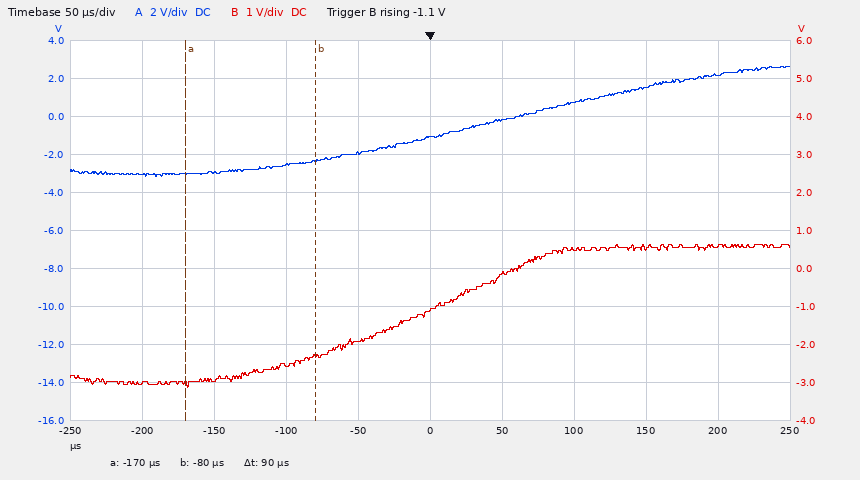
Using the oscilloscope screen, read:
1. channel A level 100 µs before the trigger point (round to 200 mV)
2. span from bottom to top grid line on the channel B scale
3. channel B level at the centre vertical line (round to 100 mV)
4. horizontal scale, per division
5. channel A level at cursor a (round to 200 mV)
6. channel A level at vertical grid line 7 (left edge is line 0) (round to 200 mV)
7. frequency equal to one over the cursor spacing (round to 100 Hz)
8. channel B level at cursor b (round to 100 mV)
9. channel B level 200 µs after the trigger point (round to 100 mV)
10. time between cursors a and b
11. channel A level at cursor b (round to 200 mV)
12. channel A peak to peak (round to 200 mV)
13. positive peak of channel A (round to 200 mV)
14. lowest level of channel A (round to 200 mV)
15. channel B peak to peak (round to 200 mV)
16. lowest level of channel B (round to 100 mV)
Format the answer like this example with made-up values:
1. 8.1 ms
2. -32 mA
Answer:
1. -2.6 V
2. 10 V
3. -1.1 V
4. 50 µs
5. -3.0 V
6. 800 mV
7. 11.1 kHz
8. -2.3 V
9. 600 mV
10. 90 µs
11. -2.4 V
12. 5.8 V
13. 2.6 V
14. -3.2 V
15. 3.8 V
16. -3.1 V
